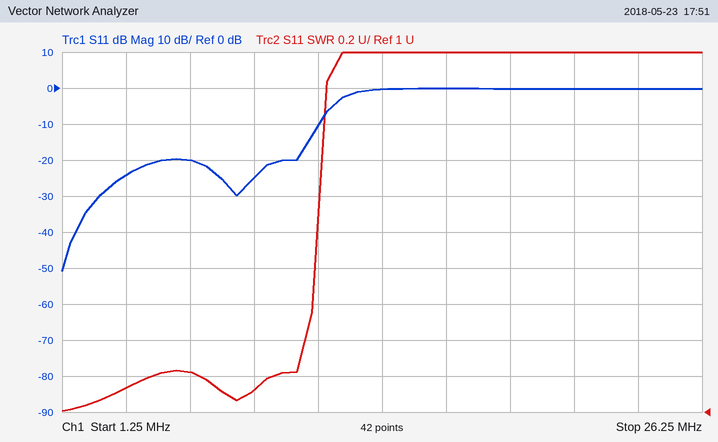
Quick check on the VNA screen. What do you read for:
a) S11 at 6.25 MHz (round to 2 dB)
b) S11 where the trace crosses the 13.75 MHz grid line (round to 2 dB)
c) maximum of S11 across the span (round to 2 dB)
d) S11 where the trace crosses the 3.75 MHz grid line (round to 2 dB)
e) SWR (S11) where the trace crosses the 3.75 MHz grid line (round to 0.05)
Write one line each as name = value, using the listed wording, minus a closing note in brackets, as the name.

S11 at 6.25 MHz = -20 dB
S11 where the trace crosses the 13.75 MHz grid line = 0 dB
maximum of S11 across the span = 0 dB
S11 where the trace crosses the 3.75 MHz grid line = -24 dB
SWR (S11) where the trace crosses the 3.75 MHz grid line = 1.15
